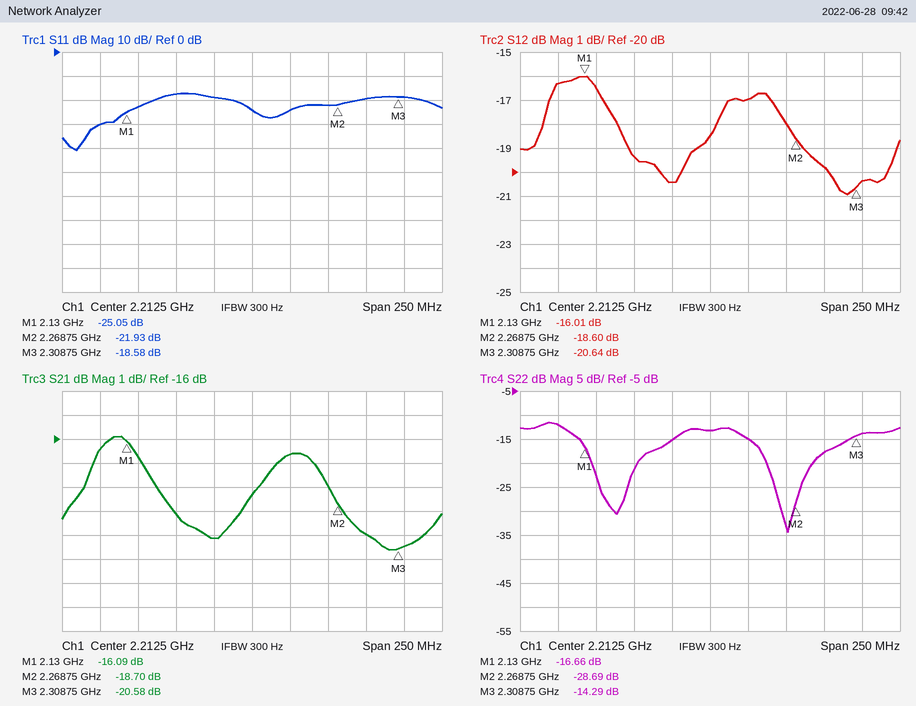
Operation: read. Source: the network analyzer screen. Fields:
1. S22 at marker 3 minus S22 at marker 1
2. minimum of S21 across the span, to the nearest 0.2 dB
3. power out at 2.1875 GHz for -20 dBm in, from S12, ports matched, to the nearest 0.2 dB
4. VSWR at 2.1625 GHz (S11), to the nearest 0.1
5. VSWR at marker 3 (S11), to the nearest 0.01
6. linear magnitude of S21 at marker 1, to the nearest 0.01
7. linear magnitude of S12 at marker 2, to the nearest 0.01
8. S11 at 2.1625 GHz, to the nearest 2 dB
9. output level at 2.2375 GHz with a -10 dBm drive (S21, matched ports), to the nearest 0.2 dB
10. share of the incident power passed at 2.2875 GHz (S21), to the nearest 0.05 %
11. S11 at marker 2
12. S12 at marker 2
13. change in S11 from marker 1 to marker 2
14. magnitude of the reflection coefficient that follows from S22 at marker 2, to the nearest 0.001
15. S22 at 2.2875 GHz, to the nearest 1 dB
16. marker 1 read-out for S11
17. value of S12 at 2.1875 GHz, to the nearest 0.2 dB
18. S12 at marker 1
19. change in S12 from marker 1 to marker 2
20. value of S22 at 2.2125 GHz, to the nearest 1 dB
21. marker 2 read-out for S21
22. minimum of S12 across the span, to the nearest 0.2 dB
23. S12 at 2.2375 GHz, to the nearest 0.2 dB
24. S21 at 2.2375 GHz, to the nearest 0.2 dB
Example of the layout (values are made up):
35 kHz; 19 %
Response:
2.37 dB; -20.6 dB; -40.4 dBm; 1.3; 1.27; 0.16; 0.12; -18 dB; -26.6 dBm; 1.00 %; -21.93 dB; -18.60 dB; 3.12 dB; 0.037; -18 dB; -25.05 dB; -20.4 dB; -16.01 dB; -2.59 dB; -13 dB; -18.70 dB; -21.0 dB; -17.0 dB; -16.6 dB
